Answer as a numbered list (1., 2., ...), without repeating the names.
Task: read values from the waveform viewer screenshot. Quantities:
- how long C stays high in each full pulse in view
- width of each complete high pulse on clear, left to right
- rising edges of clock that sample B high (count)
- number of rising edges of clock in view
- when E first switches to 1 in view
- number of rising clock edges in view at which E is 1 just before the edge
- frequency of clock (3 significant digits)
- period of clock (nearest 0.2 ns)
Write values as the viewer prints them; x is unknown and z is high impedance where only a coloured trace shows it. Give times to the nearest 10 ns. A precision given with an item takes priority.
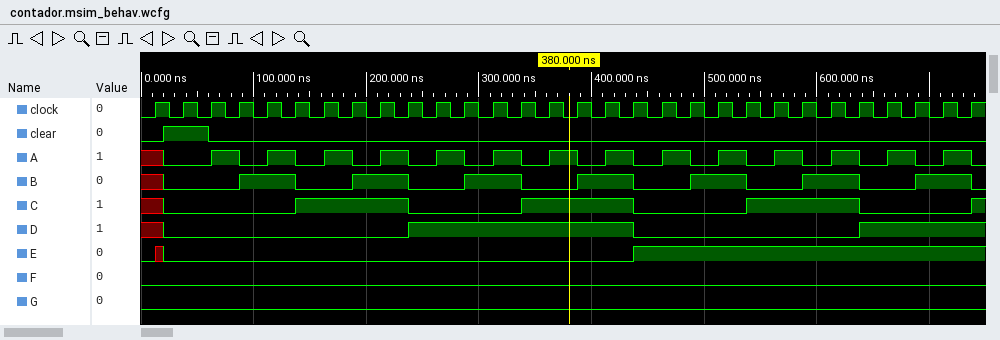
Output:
1. 100 ns, 100 ns, 100 ns
2. 40 ns
3. 14
4. 30
5. 440 ns
6. 12
7. 40.0 MHz
8. 25 ns
